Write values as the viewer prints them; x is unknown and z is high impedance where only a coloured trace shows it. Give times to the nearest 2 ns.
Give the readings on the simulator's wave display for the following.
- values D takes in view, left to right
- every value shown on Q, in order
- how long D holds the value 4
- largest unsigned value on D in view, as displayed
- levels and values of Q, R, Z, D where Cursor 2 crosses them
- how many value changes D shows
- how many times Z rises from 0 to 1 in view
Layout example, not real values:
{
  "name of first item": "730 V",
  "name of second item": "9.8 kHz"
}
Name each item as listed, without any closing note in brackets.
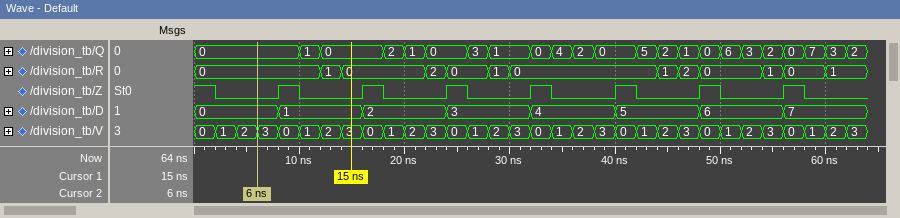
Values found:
{
  "values D takes in view, left to right": "0, 1, 2, 3, 4, 5, 6, 7",
  "every value shown on Q, in order": "0, 1, 0, 2, 1, 0, 3, 1, 0, 4, 2, 0, 5, 2, 1, 0, 6, 3, 2, 0, 7, 3, 2",
  "how long D holds the value 4": "8 ns",
  "largest unsigned value on D in view, as displayed": "7",
  "levels and values of Q, R, Z, D where Cursor 2 crosses them": "Q=0, R=0, Z=0, D=0",
  "how many value changes D shows": "7",
  "how many times Z rises from 0 to 1 in view": "7"
}
